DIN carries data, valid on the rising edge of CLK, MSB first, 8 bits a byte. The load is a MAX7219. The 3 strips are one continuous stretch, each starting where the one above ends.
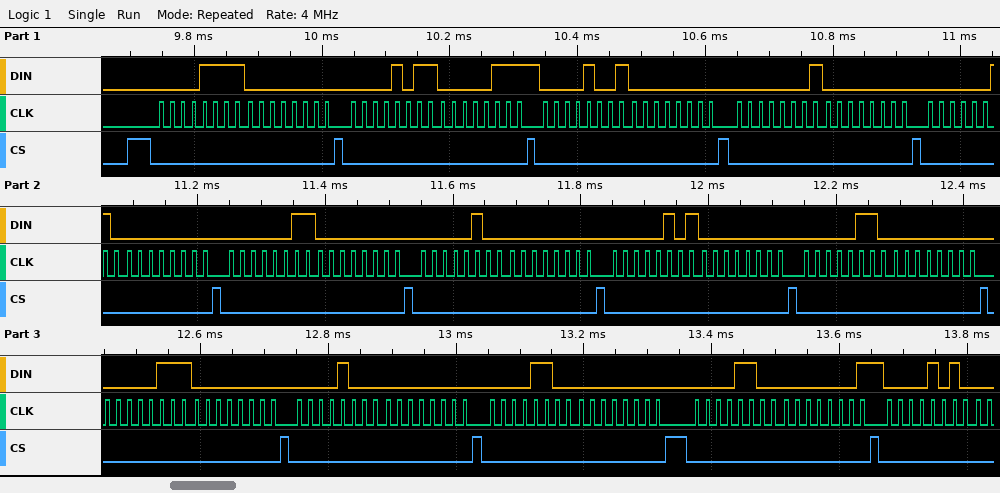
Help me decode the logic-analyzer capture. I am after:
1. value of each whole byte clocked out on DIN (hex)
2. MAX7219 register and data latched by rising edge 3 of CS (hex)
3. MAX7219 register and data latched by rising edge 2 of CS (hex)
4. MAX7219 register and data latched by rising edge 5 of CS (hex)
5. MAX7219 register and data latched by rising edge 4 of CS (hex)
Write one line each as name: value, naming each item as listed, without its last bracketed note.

value of each whole byte clocked out on DIN: 0x0F 0x00 0x0B 0x07 0x09 0x00 0x01 0x00 0x02 0x00 0x03 0x00 0x04 0x00 0x05 0x00 0x06 0x00 0x07 0x00 0x08 0x00 0x0C 0x00 0x0C 0x01 0x0A
MAX7219 register and data latched by rising edge 3 of CS: register 0xB, data 0x07
MAX7219 register and data latched by rising edge 2 of CS: register 0xF, data 0x00
MAX7219 register and data latched by rising edge 5 of CS: register 0x1, data 0x00
MAX7219 register and data latched by rising edge 4 of CS: register 0x9, data 0x00
